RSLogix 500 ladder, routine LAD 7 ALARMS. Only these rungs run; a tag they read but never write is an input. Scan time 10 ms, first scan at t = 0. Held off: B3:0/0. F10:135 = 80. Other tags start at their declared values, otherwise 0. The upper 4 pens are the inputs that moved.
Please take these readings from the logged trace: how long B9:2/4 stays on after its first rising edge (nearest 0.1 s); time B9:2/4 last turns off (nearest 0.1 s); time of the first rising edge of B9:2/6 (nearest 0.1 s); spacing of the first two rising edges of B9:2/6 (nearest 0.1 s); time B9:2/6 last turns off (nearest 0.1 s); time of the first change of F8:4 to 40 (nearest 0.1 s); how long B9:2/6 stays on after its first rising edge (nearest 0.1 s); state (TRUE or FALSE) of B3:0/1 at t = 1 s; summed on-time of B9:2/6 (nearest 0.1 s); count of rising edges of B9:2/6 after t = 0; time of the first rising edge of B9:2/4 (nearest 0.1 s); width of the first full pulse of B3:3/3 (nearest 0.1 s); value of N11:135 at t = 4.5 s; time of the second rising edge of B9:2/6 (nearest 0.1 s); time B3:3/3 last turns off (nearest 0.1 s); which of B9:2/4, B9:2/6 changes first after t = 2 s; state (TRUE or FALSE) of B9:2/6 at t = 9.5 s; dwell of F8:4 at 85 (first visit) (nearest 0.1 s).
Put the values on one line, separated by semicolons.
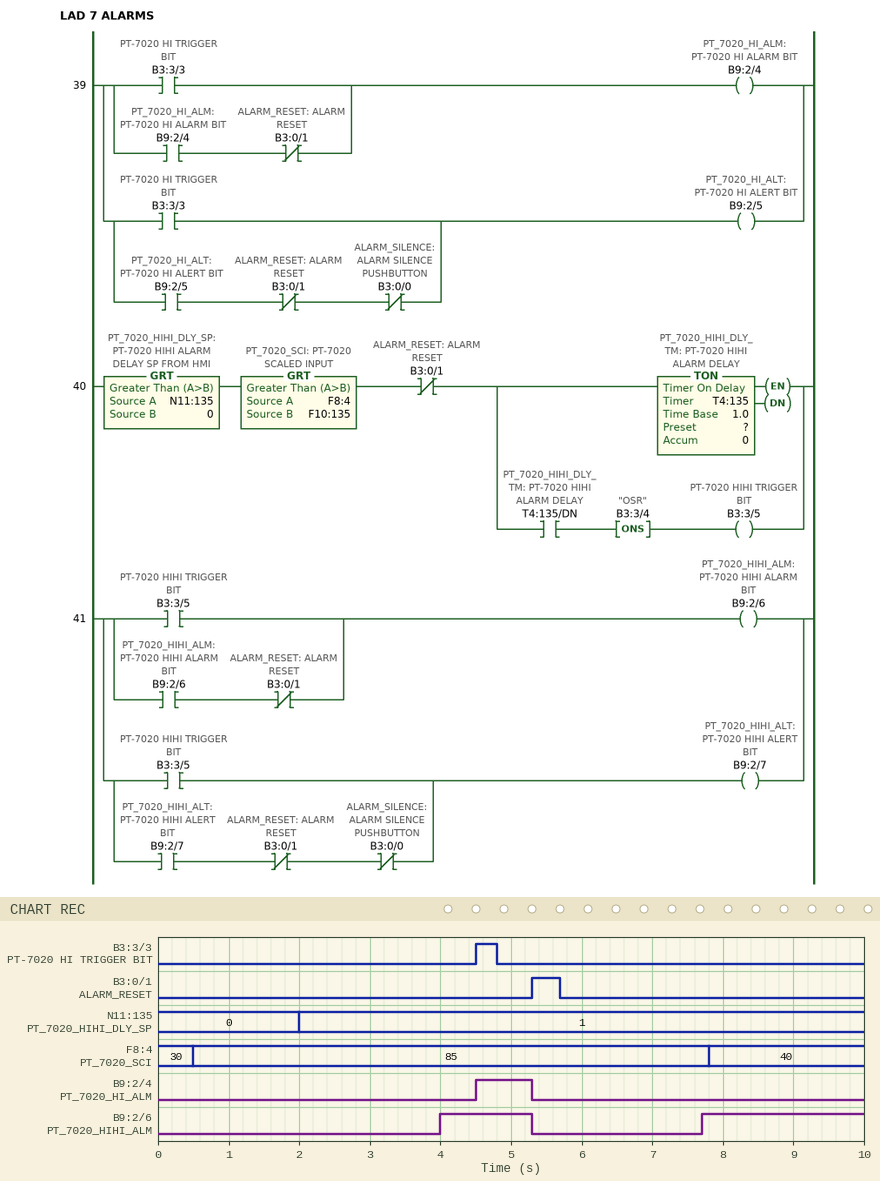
0.8 s; 5.3 s; 4.0 s; 3.7 s; 5.3 s; 7.8 s; 1.3 s; FALSE; 3.6 s; 2; 4.5 s; 0.3 s; 1; 7.7 s; 4.8 s; B9:2/6; TRUE; 7.3 s
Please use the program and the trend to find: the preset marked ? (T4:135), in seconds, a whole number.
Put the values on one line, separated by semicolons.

2 s
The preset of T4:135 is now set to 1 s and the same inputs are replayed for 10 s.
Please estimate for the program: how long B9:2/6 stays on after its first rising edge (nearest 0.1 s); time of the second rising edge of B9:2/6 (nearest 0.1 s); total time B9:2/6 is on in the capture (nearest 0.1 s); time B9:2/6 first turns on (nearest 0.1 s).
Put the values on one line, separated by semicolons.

2.3 s; 6.7 s; 5.6 s; 3.0 s
